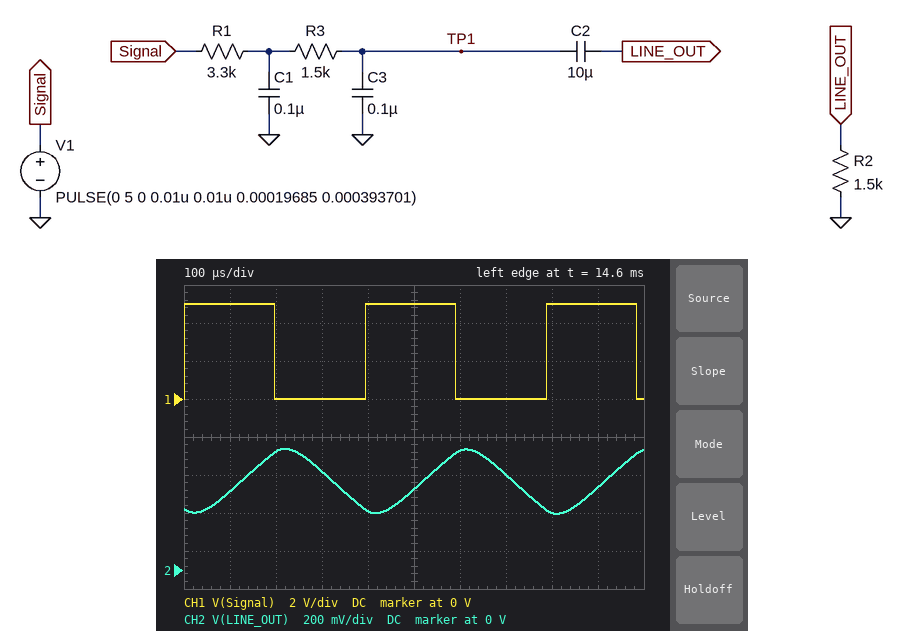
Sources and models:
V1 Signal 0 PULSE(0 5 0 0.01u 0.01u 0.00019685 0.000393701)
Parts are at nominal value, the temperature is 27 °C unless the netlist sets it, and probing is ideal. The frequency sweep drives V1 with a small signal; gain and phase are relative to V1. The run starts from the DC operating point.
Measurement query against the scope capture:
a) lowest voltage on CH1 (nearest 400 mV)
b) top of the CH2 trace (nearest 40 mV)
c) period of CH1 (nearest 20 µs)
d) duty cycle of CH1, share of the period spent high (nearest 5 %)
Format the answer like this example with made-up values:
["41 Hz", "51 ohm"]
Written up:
["0 V", "640 mV", "400 µs", "50 %"]
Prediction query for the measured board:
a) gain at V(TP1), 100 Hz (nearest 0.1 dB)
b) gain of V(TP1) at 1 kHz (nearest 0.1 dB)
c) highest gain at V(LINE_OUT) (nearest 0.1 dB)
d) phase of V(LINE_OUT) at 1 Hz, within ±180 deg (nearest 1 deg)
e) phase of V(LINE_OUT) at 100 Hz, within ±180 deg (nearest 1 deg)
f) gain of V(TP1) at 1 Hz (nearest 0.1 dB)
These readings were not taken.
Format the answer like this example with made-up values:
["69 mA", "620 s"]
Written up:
["-12.6 dB", "-17.5 dB", "-12.6 dB", "68 deg", "-8 deg", "-0.6 dB"]
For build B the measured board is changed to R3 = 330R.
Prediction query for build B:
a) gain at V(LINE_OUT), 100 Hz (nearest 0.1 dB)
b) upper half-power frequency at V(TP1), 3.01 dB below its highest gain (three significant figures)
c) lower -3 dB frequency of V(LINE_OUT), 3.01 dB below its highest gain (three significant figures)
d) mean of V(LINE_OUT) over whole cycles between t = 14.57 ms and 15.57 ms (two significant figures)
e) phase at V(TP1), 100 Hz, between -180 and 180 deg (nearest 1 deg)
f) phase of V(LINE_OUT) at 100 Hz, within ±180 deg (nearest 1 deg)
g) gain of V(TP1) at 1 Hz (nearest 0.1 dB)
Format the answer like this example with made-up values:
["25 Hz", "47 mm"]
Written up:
["-10.8 dB", "3.37 Hz", "3.05 Hz", "540 mV", "-12 deg", "-6 deg", "-0.4 dB"]
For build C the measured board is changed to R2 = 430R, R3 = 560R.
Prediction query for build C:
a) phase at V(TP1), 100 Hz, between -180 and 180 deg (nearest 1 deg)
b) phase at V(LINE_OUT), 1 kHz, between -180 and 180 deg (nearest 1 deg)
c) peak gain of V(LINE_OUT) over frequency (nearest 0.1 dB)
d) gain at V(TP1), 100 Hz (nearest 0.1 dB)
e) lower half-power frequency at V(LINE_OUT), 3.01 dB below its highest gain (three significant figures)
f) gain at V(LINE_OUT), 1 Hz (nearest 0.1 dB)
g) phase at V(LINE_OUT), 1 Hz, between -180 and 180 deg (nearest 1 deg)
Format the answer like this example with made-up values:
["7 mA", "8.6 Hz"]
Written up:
["-22 deg", "-37 deg", "-20.1 dB", "-19.6 dB", "3.64 Hz", "-31.7 dB", "75 deg"]
